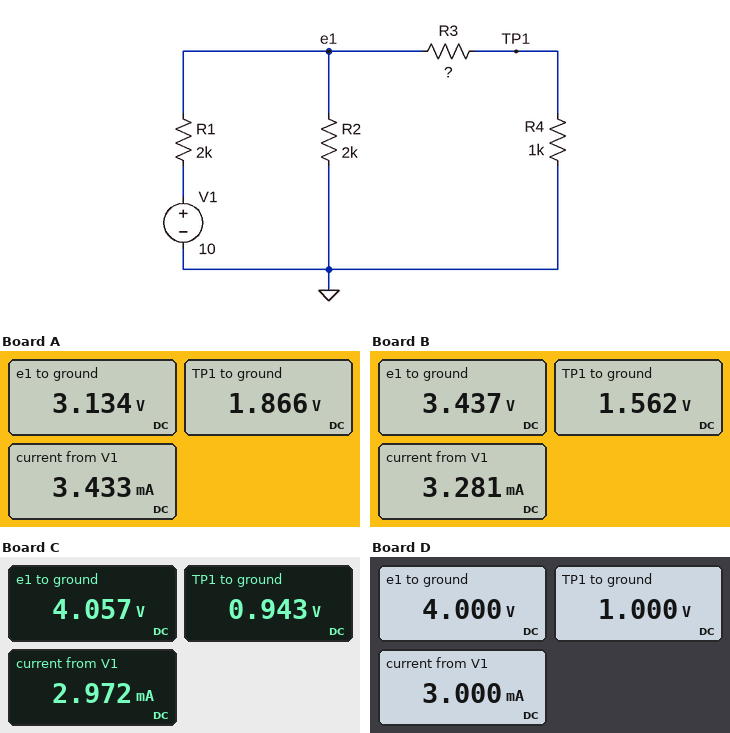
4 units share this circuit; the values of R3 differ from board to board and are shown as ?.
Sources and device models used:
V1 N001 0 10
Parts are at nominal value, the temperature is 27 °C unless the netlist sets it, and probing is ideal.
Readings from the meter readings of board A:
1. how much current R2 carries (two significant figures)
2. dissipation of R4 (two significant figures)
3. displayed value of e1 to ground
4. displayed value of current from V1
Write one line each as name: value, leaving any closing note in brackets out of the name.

how much current R2 carries: 1.6 mA
dissipation of R4: 3.5 mW
displayed value of e1 to ground: 3.134 V
displayed value of current from V1: 3.433 mA
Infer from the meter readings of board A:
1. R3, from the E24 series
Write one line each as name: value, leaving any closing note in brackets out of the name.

R3, from the E24 series: 680 Ω
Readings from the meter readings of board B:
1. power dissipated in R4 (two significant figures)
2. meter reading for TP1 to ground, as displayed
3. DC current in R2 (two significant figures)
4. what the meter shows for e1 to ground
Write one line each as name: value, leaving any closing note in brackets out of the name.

power dissipated in R4: 2.4 mW
meter reading for TP1 to ground, as displayed: 1.562 V
DC current in R2: 1.7 mA
what the meter shows for e1 to ground: 3.437 V
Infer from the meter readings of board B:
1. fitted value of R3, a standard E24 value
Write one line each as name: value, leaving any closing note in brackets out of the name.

fitted value of R3, a standard E24 value: 1.2 kΩ
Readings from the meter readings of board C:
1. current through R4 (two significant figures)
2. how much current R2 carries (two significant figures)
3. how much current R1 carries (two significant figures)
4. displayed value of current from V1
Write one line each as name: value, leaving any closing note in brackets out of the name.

current through R4: 940 µA
how much current R2 carries: 2.0 mA
how much current R1 carries: 3.0 mA
displayed value of current from V1: 2.972 mA
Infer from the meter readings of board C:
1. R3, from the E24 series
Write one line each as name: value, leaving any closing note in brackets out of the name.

R3, from the E24 series: 3.3 kΩ
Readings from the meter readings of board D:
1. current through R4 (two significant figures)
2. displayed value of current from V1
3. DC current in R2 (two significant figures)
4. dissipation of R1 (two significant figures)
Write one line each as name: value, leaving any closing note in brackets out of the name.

current through R4: 1.0 mA
displayed value of current from V1: 3.000 mA
DC current in R2: 2.0 mA
dissipation of R1: 18 mW
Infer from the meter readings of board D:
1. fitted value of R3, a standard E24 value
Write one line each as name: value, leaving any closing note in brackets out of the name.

fitted value of R3, a standard E24 value: 3 kΩ
